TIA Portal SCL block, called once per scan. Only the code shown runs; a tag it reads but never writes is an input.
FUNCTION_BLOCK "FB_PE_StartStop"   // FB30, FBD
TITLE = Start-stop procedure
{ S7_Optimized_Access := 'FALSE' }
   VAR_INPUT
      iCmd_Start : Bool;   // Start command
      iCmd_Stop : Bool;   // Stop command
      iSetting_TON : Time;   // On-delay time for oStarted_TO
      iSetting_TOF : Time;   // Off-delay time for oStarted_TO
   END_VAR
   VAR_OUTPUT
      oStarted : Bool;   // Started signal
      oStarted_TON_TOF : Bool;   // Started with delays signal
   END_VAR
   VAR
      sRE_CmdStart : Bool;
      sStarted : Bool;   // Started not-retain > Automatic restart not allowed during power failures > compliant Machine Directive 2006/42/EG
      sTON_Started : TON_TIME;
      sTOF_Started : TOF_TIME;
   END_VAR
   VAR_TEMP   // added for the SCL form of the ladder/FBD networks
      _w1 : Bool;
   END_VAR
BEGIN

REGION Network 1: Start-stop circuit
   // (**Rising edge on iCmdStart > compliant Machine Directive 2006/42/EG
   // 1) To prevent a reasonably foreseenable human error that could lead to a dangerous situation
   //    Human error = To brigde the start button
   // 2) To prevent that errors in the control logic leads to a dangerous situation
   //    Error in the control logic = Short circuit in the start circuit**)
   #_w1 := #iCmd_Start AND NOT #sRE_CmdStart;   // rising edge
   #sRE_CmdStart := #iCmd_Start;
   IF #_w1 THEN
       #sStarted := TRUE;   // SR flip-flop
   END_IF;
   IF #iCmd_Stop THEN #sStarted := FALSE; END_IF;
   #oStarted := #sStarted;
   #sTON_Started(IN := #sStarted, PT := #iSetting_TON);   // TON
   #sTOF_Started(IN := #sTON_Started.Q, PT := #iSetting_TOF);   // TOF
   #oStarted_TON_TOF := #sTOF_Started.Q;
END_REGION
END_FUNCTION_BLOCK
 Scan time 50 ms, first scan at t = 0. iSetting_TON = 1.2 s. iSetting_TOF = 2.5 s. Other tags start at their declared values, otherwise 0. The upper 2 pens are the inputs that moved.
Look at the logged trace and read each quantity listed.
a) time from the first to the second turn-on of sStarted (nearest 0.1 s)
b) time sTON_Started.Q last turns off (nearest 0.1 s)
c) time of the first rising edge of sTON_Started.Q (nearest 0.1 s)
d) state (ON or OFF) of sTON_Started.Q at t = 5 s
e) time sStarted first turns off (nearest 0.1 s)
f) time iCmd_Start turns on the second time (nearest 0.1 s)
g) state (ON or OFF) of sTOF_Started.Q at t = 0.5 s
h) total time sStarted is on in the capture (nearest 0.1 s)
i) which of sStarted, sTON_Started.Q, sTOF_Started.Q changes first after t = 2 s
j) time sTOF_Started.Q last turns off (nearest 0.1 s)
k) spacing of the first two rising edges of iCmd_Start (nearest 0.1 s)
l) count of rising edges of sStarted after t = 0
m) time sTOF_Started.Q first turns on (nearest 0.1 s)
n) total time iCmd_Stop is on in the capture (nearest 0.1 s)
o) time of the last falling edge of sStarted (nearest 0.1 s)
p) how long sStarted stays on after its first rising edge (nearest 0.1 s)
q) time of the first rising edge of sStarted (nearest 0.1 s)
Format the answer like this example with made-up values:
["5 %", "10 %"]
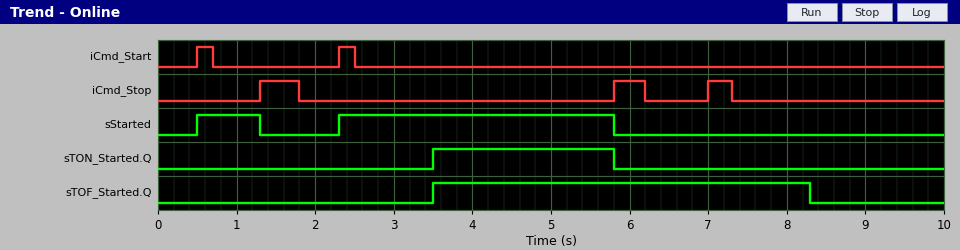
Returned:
["1.8 s", "5.8 s", "3.5 s", "ON", "1.3 s", "2.3 s", "OFF", "4.3 s", "sStarted", "8.3 s", "1.8 s", "2", "3.5 s", "1.2 s", "5.8 s", "0.8 s", "0.5 s"]
